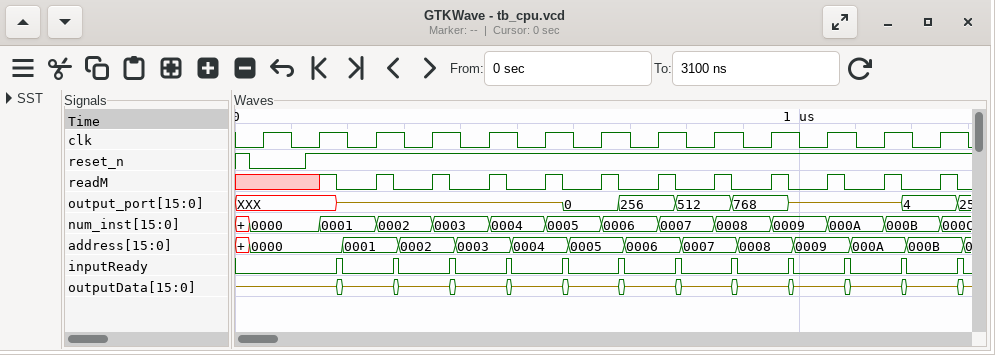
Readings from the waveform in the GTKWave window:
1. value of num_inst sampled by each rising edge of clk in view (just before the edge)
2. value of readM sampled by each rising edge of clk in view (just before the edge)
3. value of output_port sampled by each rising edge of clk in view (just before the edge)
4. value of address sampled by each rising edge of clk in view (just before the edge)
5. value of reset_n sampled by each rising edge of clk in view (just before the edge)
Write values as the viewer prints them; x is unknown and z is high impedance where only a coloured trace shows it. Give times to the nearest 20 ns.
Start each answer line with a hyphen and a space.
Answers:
- 0000, 0000, 0001, 0002, 0003, 0004, 0005, 0006, 0007, 0008, 0009, 000A, 000B
- x x 0 0 0 0 0 0 0 0 0 0 0
- XXX, XXX, z, z, z, z, 0, 256, 512, 768, z, z, 4
- 0000, 0000, 0001, 0002, 0003, 0004, 0005, 0006, 0007, 0008, 0009, 000A, 000B
- 0 1 1 1 1 1 1 1 1 1 1 1 1
